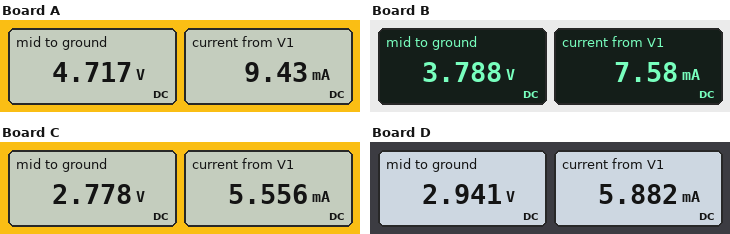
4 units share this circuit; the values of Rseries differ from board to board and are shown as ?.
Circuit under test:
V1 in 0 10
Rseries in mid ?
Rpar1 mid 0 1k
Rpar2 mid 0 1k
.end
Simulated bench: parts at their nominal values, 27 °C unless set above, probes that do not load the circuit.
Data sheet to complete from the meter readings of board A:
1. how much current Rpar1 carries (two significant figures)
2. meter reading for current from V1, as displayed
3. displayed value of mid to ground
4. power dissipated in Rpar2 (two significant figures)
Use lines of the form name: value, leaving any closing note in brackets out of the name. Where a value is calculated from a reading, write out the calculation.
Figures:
how much current Rpar1 carries: (4.717 V) / 1 kΩ = 4.7 mA
meter reading for current from V1, as displayed: 9.43 mA
displayed value of mid to ground: 4.717 V
power dissipated in Rpar2: (4.717 V)^2 / 1 kΩ = 22 mW
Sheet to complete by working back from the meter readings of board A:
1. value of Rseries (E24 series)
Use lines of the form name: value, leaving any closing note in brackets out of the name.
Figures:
value of Rseries: 560 Ω
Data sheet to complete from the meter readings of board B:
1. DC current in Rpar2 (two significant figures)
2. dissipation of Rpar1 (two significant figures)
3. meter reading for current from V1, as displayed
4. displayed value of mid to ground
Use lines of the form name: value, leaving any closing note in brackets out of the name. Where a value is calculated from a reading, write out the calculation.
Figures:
DC current in Rpar2: (3.788 V) / 1 kΩ = 3.8 mA
dissipation of Rpar1: (3.788 V)^2 / 1 kΩ = 14 mW
meter reading for current from V1, as displayed: 7.58 mA
displayed value of mid to ground: 3.788 V
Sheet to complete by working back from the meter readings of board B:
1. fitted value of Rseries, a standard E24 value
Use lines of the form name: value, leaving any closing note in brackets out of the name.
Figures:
fitted value of Rseries, a standard E24 value: 820 Ω
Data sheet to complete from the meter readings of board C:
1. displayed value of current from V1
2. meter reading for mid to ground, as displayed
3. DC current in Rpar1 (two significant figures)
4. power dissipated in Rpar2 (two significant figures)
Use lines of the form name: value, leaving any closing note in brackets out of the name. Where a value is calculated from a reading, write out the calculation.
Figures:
displayed value of current from V1: 5.556 mA
meter reading for mid to ground, as displayed: 2.778 V
DC current in Rpar1: (2.778 V) / 1 kΩ = 2.8 mA
power dissipated in Rpar2: (2.778 V)^2 / 1 kΩ = 7.7 mW
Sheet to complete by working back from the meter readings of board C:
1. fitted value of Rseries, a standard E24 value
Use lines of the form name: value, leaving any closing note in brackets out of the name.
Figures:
fitted value of Rseries, a standard E24 value: 1.3 kΩ
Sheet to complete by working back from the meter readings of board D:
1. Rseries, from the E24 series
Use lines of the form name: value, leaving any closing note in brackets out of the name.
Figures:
Rseries, from the E24 series: 1.2 kΩ
